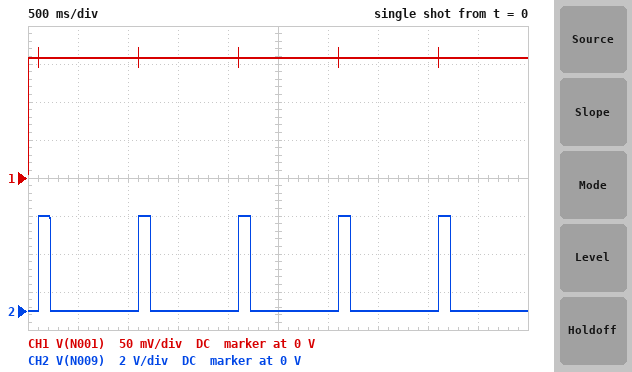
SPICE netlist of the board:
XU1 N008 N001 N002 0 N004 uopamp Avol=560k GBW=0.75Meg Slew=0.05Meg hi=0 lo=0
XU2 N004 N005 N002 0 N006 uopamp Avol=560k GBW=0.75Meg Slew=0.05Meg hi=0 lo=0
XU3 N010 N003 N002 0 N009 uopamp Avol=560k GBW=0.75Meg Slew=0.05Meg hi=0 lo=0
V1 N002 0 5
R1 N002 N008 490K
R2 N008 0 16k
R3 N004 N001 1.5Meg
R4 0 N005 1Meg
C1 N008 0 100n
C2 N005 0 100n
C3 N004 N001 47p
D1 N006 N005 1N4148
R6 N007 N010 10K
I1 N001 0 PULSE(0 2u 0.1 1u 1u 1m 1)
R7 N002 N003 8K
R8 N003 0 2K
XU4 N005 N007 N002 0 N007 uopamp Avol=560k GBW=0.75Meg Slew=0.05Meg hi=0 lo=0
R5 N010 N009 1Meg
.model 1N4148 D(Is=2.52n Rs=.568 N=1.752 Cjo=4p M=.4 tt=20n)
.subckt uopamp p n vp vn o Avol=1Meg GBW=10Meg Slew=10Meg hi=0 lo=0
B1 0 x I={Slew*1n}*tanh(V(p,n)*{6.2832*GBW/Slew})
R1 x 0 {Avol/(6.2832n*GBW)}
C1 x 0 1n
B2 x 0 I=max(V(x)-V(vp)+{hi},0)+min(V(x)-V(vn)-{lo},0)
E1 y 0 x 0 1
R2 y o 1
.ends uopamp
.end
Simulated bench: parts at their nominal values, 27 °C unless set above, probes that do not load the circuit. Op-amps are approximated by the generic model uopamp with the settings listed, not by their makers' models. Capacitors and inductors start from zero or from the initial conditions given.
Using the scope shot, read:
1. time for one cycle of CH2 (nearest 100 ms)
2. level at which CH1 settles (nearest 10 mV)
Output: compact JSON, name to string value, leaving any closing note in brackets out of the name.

{"time for one cycle of CH2": "1.0 s", "level at which CH1 settles": "160 mV"}
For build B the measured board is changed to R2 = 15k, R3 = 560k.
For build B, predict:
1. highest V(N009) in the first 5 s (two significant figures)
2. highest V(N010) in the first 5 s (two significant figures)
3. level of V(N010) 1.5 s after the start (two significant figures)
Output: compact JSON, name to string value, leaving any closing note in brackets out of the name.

{"highest V(N009) in the first 5 s": "5.0 V", "highest V(N010) in the first 5 s": "1.3 V", "level of V(N010) 1.5 s after the start": "150 mV"}
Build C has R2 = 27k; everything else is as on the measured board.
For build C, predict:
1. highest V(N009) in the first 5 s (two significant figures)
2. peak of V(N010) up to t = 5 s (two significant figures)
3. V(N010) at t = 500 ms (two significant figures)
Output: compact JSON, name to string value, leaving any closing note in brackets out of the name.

{"highest V(N009) in the first 5 s": "5.0 V", "peak of V(N010) up to t = 5 s": "3.3 V", "V(N010) at t = 500 ms": "260 mV"}
